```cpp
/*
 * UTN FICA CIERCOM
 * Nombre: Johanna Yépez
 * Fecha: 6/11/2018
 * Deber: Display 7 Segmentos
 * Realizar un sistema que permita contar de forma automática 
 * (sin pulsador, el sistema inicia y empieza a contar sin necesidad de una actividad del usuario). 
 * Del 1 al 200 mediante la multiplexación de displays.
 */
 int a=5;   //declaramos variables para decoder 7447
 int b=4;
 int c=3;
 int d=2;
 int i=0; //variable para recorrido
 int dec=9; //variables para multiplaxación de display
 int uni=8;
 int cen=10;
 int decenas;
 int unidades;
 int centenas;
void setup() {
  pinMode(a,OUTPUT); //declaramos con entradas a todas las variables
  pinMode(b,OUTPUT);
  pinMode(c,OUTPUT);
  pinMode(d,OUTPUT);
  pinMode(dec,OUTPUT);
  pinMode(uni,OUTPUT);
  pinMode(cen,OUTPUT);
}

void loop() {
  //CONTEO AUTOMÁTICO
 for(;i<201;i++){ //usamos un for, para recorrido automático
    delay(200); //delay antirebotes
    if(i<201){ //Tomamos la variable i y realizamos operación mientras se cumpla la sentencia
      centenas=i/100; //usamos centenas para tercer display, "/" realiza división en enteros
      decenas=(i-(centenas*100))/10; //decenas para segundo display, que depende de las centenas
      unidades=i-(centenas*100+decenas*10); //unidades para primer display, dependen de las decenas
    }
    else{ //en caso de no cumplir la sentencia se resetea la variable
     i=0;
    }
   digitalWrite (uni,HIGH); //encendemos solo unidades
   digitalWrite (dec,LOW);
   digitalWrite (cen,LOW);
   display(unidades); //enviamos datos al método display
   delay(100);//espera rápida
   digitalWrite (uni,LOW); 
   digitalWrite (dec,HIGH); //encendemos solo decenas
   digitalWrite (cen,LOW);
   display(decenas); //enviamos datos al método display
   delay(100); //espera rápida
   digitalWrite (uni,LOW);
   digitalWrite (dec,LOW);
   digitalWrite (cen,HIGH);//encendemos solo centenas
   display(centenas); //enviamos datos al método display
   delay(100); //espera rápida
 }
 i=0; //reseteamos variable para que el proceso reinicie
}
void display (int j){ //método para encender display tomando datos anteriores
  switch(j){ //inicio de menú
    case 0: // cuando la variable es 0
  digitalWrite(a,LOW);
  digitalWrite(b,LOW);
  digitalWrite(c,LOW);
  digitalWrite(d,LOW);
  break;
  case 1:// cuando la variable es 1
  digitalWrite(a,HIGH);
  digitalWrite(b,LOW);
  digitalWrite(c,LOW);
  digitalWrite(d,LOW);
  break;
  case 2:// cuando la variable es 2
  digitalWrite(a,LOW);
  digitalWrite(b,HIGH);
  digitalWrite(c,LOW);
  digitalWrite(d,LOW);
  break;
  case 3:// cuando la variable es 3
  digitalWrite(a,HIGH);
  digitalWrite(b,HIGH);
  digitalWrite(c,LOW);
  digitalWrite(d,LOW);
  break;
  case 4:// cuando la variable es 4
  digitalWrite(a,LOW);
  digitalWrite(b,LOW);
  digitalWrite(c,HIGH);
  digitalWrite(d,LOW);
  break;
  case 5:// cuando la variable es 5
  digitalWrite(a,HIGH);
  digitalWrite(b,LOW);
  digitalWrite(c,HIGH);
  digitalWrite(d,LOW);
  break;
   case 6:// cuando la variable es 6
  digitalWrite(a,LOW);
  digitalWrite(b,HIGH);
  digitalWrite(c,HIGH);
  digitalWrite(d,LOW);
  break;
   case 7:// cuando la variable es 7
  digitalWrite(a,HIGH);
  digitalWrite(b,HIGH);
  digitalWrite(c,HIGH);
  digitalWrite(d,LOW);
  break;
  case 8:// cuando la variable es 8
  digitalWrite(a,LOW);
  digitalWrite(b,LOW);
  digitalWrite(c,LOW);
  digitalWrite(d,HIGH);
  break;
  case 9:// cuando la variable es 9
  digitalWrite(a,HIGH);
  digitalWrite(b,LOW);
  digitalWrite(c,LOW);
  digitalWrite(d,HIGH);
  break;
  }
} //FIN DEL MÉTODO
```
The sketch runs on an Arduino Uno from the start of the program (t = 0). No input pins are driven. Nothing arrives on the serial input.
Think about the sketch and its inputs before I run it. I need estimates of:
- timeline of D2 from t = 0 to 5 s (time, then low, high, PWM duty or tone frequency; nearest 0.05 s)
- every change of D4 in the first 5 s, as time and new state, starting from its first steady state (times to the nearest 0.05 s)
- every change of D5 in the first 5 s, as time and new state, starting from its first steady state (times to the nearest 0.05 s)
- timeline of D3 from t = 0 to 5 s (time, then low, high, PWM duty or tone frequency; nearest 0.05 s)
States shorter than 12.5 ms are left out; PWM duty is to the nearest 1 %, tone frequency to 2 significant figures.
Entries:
0 s low; 4.2 s high; 4.3 s low; 4.7 s high; 4.8 s low
0 s low; 1.2 s high; 1.3 s low; 1.7 s high; 1.8 s low; 3.2 s high; 3.3 s low; 3.7 s high; 3.8 s low
0 s low; 0.7 s high; 0.8 s low; 1.7 s high; 1.8 s low; 2.7 s high; 2.8 s low; 3.7 s high; 3.8 s low; 4.7 s high; 4.8 s low
0 s low; 2.2 s high; 2.3 s low; 2.7 s high; 2.8 s low; 3.2 s high; 3.3 s low; 3.7 s high; 3.8 s low
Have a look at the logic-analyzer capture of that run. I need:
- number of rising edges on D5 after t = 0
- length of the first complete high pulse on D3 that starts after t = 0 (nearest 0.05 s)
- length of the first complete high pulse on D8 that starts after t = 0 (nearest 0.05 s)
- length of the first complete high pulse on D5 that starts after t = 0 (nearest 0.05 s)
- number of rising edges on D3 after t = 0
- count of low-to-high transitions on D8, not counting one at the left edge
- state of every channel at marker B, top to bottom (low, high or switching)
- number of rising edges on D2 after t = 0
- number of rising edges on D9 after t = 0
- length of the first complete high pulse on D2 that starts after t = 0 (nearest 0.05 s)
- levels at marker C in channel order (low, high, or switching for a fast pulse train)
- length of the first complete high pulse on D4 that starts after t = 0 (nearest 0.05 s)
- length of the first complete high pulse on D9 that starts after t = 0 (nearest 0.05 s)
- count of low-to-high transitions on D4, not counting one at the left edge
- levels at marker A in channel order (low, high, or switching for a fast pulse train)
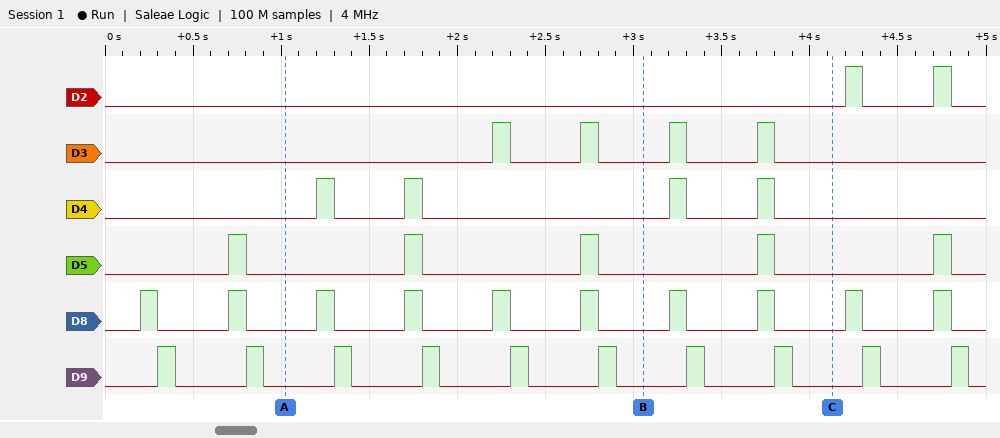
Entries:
5
0.10 s
0.10 s
0.10 s
4
10
D2 low, D3 low, D4 low, D5 low, D8 low, D9 low
2
10
0.10 s
D2 low, D3 low, D4 low, D5 low, D8 low, D9 low
0.10 s
0.10 s
4
D2 low, D3 low, D4 low, D5 low, D8 low, D9 low
